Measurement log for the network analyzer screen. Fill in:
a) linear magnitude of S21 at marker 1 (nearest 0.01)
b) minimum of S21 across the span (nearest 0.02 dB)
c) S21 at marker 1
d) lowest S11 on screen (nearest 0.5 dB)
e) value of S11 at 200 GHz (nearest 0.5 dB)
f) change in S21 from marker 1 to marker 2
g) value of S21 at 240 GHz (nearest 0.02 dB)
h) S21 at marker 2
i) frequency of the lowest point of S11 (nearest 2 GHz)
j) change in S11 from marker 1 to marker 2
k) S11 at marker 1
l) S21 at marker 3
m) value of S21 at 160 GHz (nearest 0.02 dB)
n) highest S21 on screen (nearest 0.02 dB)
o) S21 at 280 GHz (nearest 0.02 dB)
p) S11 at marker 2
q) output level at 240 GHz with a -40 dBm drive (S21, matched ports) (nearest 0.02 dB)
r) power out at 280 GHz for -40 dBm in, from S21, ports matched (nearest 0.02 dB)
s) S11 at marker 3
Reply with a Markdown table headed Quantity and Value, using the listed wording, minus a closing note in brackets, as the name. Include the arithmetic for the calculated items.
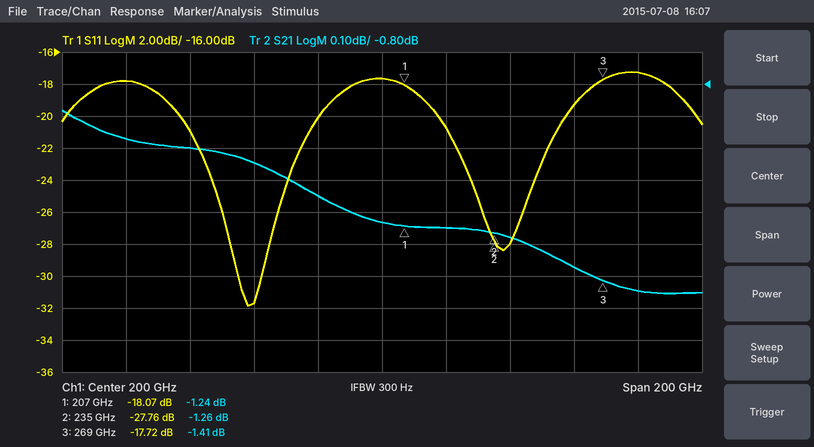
| Quantity | Value |
|---|---|
| linear magnitude of S21 at marker 1 | 10^(-1.24/20) ≈ 0.87 |
| minimum of S21 across the span | -1.46 dB |
| S21 at marker 1 | -1.24 dB |
| lowest S11 on screen | -32.0 dB |
| value of S11 at 200 GHz | -17.5 dB |
| change in S21 from marker 1 to marker 2 | -1.26 − (-1.24) = -0.02 dB |
| value of S21 at 240 GHz | -1.28 dB |
| S21 at marker 2 | -1.26 dB |
| frequency of the lowest point of S11 | 158 GHz |
| change in S11 from marker 1 to marker 2 | -27.76 − (-18.07) = -9.69 dB |
| S11 at marker 1 | -18.07 dB |
| S21 at marker 3 | -1.41 dB |
| value of S21 at 160 GHz | -1.04 dB |
| highest S21 on screen | -0.88 dB |
| S21 at 280 GHz | -1.44 dB |
| S11 at marker 2 | -27.76 dB |
| output level at 240 GHz with a -40 dBm drive (S21, matched ports) | -40 dBm + (-1.28 dB) = -41.28 dBm |
| power out at 280 GHz for -40 dBm in, from S21, ports matched | -40 dBm + (-1.44 dB) = -41.44 dBm |
| S11 at marker 3 | -17.72 dB |
